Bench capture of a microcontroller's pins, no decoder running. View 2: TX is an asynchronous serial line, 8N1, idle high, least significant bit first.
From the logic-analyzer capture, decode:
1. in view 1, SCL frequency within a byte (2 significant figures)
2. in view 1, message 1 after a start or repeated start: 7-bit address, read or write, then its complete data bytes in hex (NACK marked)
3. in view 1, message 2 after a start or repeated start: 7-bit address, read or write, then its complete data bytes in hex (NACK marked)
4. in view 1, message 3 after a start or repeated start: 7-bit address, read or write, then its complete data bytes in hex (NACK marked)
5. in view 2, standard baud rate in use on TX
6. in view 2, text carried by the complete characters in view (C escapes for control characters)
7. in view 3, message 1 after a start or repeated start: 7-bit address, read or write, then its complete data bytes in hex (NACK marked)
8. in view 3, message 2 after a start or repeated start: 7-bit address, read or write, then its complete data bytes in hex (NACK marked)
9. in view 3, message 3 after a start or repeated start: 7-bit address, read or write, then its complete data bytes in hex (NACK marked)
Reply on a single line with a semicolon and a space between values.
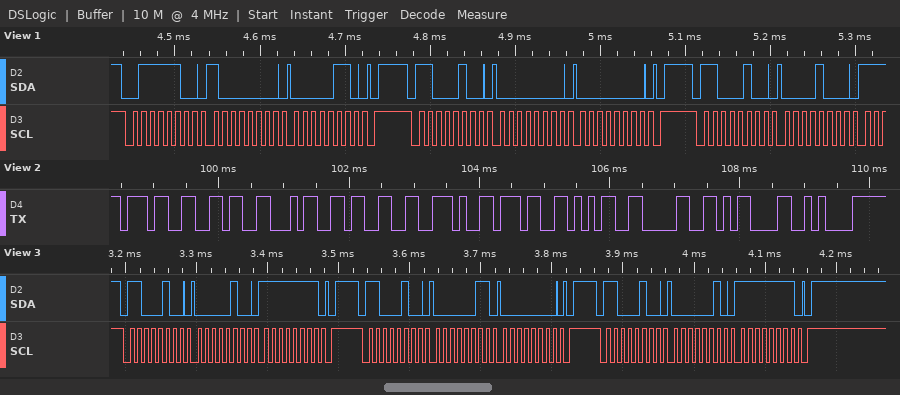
100 kHz; 0x3E write: 80 06; 0x62 write: 00 00; 0x62 write: 08; 9600 baud; "7643.750\r\n"; 0x62 write: 04 FF; 0x62 write: 03 00; 0x62 write: 02 FF
